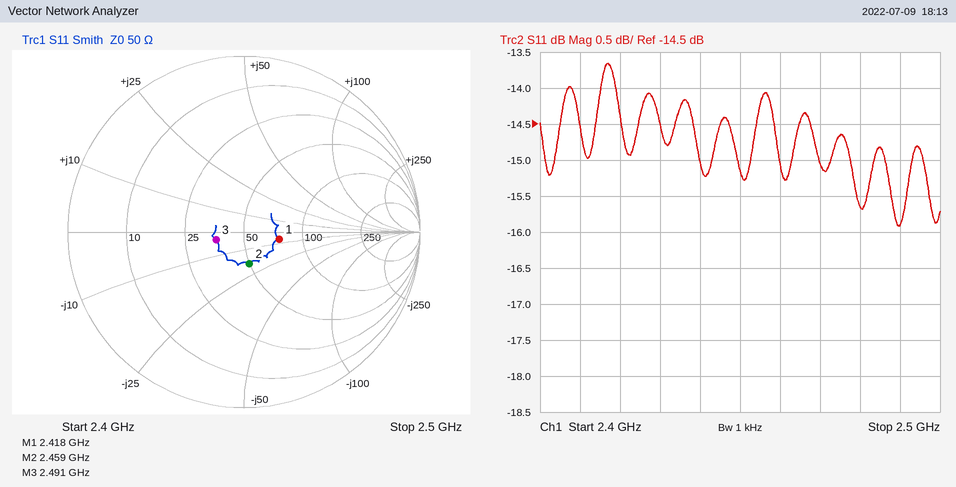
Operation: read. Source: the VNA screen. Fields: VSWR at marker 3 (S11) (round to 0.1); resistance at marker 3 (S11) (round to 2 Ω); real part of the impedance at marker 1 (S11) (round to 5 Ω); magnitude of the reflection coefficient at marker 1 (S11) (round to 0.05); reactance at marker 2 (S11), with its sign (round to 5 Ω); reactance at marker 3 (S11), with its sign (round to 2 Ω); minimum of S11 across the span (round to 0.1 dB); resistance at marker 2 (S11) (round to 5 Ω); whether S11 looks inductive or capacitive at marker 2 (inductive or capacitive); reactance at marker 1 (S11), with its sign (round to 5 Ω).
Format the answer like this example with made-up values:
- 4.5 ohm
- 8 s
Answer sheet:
- 1.4
- 36 Ω
- 75 Ω
- 0.20
- -20 Ω
- -4 Ω
- -15.9 dB
- 50 Ω
- capacitive
- -5 Ω
